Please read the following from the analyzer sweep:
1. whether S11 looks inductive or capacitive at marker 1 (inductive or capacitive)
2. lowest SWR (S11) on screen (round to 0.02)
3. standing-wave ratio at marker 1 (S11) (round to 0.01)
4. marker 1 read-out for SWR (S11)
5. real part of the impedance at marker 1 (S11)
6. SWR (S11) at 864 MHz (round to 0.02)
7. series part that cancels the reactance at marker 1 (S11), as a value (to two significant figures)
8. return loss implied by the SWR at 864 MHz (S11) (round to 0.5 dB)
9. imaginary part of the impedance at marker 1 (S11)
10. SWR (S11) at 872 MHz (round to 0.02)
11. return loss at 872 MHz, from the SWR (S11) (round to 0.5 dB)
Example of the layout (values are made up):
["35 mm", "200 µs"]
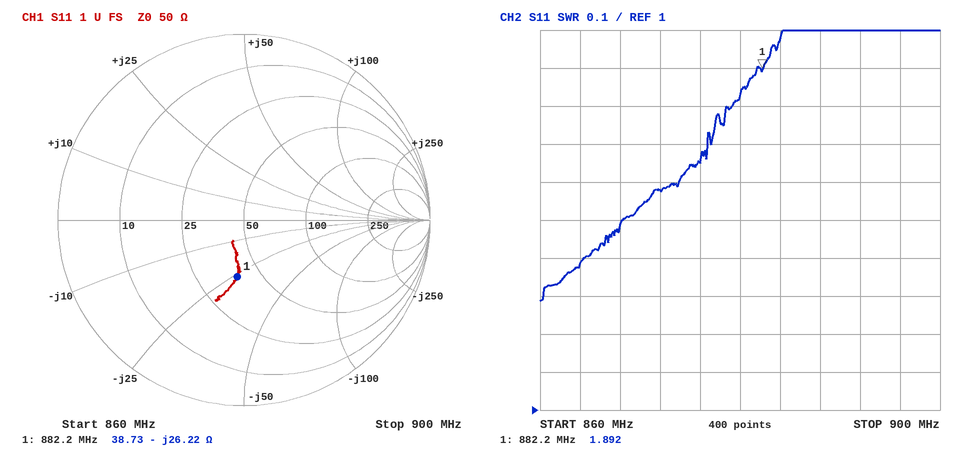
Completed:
["capacitive", "1.28", "1.89", "1.892", "38.73 Ω", "1.38", "4.7 nH", "16.0 dB", "-26.22 Ω", "1.58", "13.0 dB"]
